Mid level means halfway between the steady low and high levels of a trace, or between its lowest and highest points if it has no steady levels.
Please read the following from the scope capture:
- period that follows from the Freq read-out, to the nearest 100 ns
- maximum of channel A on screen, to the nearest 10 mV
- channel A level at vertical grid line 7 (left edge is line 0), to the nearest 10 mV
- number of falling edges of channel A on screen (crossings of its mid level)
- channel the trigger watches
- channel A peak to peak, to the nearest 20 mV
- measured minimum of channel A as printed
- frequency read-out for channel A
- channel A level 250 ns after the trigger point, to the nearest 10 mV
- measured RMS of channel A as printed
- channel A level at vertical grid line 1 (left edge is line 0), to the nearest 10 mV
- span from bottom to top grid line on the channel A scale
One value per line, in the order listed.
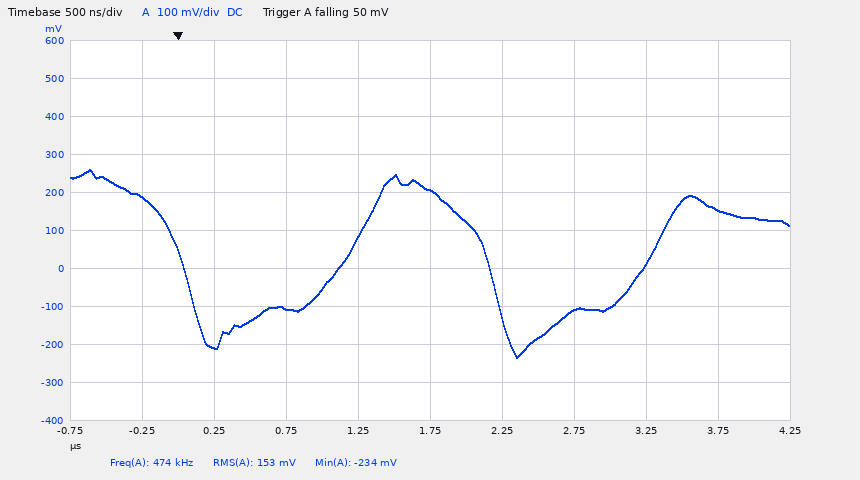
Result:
2.1 µs
260 mV
-110 mV
2
channel A
500 mV
-234 mV
474 kHz
-210 mV
153 mV
190 mV
1 V
